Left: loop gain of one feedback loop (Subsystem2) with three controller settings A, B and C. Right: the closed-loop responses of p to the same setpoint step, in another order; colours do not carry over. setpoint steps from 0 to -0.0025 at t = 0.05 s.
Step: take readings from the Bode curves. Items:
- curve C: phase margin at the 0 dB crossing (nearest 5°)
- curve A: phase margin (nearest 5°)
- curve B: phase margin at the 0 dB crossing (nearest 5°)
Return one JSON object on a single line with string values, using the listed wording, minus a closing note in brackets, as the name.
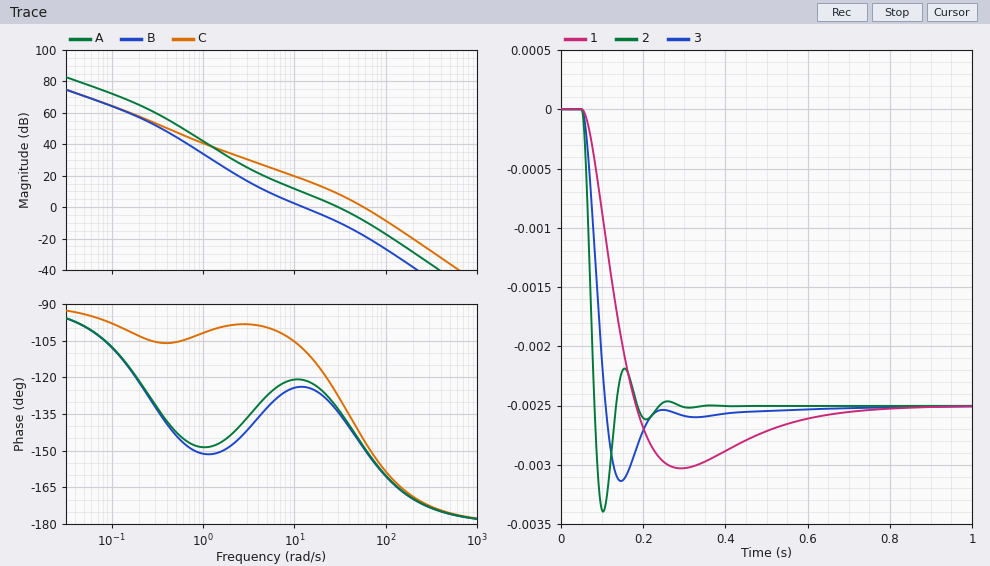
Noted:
{"curve C: phase margin at the 0 dB crossing": "35°", "curve A: phase margin": "45°", "curve B: phase margin at the 0 dB crossing": "55°"}
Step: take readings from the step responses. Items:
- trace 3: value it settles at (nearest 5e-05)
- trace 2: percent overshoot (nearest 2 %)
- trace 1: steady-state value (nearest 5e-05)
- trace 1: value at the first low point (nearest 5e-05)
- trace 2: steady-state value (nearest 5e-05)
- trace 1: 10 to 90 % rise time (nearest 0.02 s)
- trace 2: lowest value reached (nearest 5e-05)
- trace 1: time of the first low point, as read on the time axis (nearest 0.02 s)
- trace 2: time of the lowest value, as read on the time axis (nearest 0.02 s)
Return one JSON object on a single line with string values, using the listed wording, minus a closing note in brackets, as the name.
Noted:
{"trace 3: value it settles at": "-0.00250", "trace 2: percent overshoot": "36 %", "trace 1: steady-state value": "-0.00250", "trace 1: value at the first low point": "-0.00305", "trace 2: steady-state value": "-0.00250", "trace 1: 10 to 90 % rise time": "0.10 s", "trace 2: lowest value reached": "-0.00340", "trace 1: time of the first low point, as read on the time axis": "0.30 s", "trace 2: time of the lowest value, as read on the time axis": "0.10 s"}
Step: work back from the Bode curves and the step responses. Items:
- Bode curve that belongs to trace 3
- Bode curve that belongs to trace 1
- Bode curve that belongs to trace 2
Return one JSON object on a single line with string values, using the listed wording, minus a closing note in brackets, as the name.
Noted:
{"Bode curve that belongs to trace 3": "A", "Bode curve that belongs to trace 1": "B", "Bode curve that belongs to trace 2": "C"}
